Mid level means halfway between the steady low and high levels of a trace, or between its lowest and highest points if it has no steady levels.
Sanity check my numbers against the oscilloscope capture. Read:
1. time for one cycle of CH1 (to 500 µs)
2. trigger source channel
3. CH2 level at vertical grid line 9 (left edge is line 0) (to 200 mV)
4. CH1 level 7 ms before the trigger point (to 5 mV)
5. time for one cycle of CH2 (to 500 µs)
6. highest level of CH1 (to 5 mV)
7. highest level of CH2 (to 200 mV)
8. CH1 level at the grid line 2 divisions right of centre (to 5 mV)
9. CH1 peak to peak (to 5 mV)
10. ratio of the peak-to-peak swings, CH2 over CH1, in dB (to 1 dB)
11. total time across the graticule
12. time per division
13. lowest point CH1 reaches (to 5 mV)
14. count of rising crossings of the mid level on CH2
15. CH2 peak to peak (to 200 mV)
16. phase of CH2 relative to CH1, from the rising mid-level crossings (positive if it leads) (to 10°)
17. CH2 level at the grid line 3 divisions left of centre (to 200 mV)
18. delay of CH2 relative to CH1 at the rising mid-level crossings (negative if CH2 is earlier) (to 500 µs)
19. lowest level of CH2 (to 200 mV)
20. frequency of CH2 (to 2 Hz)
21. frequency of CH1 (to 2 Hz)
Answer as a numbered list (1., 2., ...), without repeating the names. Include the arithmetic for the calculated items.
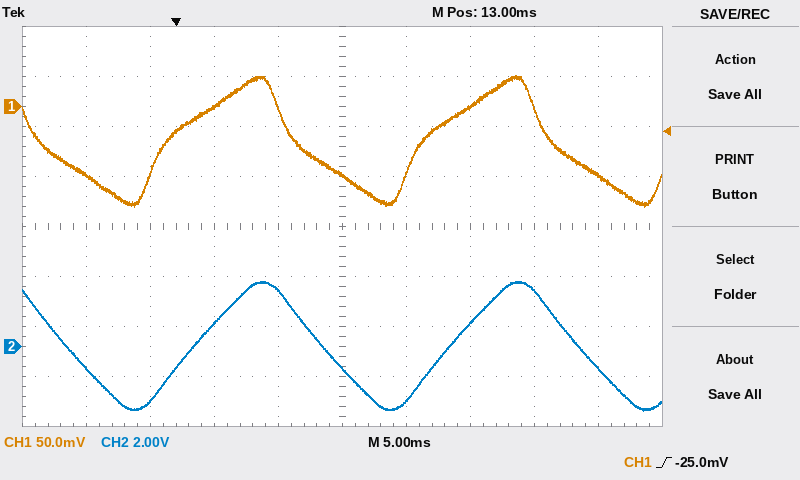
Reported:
1. 20.0 ms
2. CH1
3. -800 mV
4. -70 mV
5. 20.0 ms
6. 30 mV
7. 2.6 V
8. 0 mV
9. 30 mV − (-100 mV) = 130 mV
10. 20 log10(5.2 V / 130 mV) ≈ 32 dB
11. 50 ms
12. 5 ms
13. -100 mV
14. 2
15. 2.6 V − (-2.6 V) = 5.2 V
16. −360° × (+2.0 ms) / 20.0 ms ≈ -36.0°, so -40° to the nearest 10°
17. -2.2 V
18. +2.0 ms
19. -2.6 V
20. 1 / 20.0 ms ≈ 50 Hz
21. 1 / 20.0 ms ≈ 50 Hz
